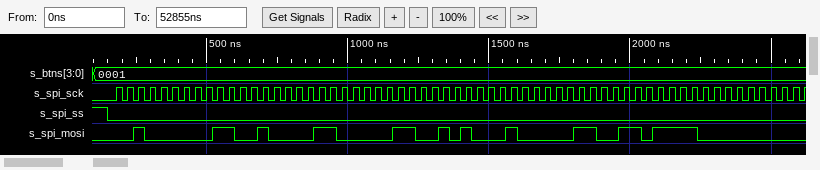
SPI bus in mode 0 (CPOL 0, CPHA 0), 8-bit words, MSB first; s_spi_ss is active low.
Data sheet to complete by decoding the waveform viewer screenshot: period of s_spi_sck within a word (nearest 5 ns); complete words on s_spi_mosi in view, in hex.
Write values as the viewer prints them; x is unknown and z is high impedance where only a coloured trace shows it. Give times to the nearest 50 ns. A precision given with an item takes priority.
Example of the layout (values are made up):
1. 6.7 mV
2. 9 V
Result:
1. 40 ns
2. 20, 64, 30, 65, 10, 66, F0
